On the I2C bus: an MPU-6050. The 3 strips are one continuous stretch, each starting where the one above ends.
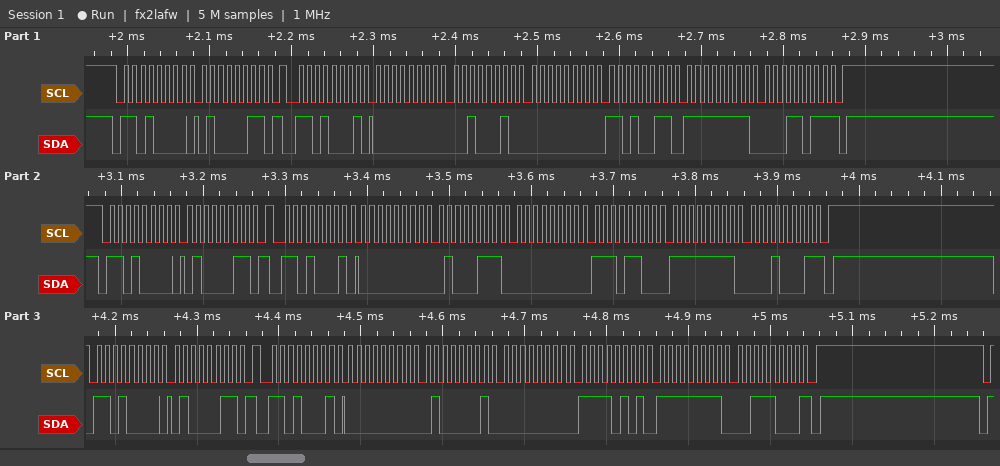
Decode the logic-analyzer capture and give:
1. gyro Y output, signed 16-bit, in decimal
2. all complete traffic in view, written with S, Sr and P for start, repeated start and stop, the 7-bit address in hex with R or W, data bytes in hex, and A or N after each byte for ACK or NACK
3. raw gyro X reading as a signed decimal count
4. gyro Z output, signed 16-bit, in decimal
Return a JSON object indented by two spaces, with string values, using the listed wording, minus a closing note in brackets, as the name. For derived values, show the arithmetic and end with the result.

{
  "gyro Y output, signed 16-bit, in decimal": "0x00D3 = 211",
  "all complete traffic in view, written with S, Sr and P for start, repeated start and stop, the 7-bit address in hex with R or W, data bytes in hex, and A or N after each byte for ACK or NACK": "S 68W A 43 A Sr 68R A 00 A 22 A 00 A D3 A FF A 1B N P S 68W A 43 A Sr 68R A 00 A 47 A 00 A EC A FF A 11 N P S 68W A 43 A Sr 68R A 00 A 41 A 00 A F5 A FF A 38 N P",
  "raw gyro X reading as a signed decimal count": "0x0022 = 34",
  "gyro Z output, signed 16-bit, in decimal": "0xFF1B = -229"
}
